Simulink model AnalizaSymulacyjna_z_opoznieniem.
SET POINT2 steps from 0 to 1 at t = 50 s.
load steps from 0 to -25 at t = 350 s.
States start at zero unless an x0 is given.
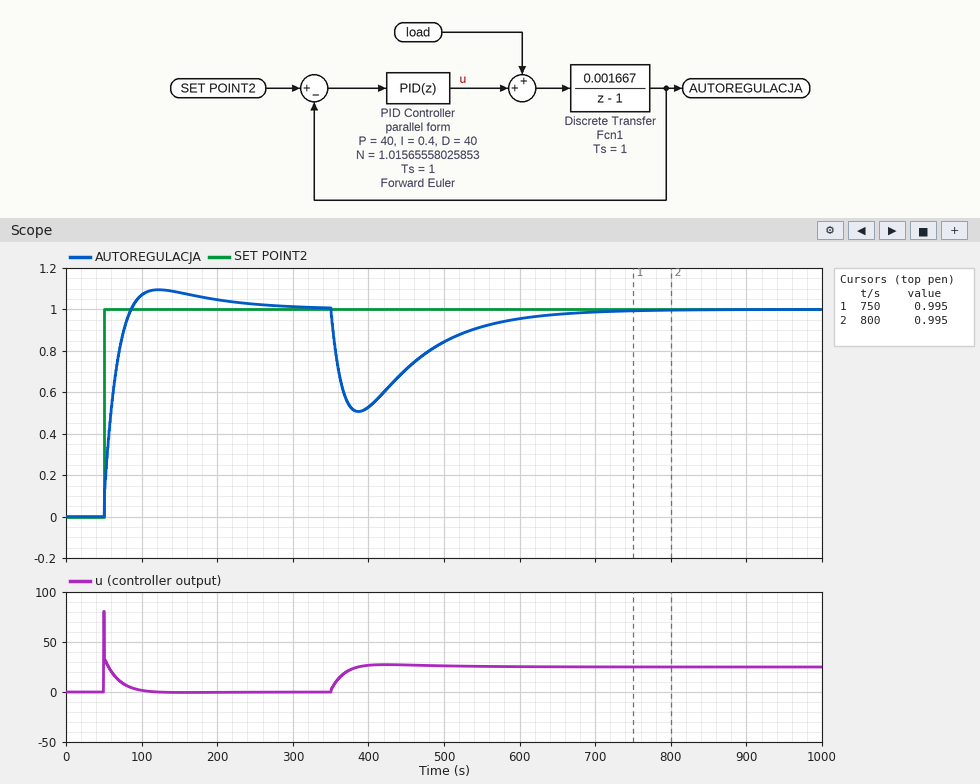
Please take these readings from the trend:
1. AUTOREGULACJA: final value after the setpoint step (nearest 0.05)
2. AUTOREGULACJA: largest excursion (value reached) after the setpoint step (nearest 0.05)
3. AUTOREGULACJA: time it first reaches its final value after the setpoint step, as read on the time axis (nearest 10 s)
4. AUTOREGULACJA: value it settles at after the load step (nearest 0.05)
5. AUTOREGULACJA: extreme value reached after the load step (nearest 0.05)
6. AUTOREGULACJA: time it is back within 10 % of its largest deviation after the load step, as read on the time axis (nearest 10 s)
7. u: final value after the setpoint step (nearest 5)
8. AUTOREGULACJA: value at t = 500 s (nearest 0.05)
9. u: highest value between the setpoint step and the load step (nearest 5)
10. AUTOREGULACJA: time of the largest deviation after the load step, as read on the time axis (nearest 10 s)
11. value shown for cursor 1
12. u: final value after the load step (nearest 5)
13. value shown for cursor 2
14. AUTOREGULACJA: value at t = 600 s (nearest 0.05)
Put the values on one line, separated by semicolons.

1.00; 1.10; 90 s; 1.00; 0.50; 590 s; 0; 0.85; 80; 390 s; 0.995; 25; 0.995; 0.95
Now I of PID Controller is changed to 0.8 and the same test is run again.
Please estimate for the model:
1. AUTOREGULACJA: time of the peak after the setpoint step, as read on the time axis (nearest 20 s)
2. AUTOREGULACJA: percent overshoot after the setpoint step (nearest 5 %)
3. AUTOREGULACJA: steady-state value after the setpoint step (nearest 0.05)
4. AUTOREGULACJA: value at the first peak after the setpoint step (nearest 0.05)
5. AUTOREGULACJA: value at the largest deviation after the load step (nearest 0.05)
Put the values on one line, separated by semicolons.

100 s; 15 %; 1.00; 1.15; 0.55
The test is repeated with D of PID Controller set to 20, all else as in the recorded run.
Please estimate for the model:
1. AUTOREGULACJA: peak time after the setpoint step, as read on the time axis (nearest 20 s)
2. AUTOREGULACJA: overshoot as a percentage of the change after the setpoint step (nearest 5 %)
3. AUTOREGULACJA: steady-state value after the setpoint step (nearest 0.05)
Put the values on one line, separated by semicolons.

120 s; 10 %; 1.00
